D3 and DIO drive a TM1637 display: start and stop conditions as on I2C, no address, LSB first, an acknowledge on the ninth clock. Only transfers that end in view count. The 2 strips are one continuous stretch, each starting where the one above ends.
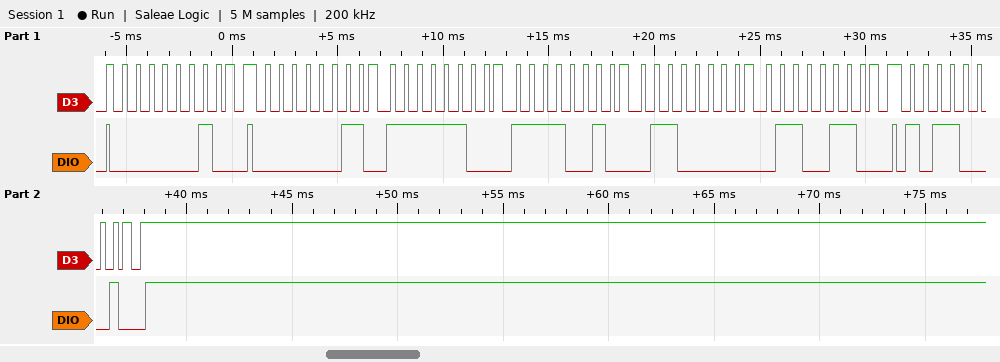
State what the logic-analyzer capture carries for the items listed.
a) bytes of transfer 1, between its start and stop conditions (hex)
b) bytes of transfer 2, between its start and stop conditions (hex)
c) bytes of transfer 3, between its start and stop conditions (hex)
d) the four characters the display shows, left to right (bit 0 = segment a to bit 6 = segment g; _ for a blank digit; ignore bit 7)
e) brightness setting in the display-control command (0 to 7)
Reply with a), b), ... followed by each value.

a) 40
b) C0 3F 4F 06 66
c) 8D
d) 0314
e) 5
